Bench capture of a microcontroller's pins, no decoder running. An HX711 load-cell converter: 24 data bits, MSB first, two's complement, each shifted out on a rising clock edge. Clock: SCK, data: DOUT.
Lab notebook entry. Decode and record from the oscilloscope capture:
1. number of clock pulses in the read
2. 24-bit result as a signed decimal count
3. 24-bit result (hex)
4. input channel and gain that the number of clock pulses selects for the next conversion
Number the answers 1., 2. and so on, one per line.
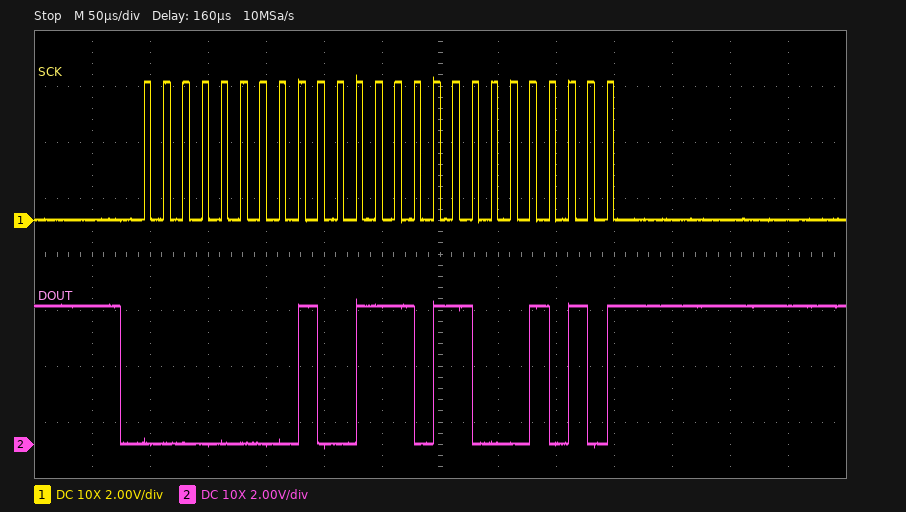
1. 25
2. 40330
3. 0x009D8A
4. channel A, gain 128
